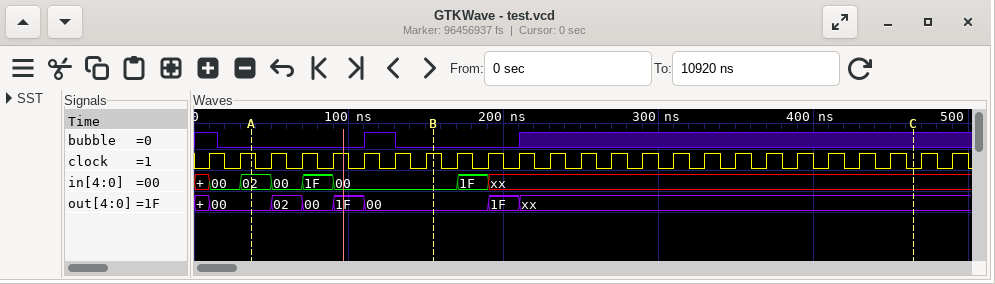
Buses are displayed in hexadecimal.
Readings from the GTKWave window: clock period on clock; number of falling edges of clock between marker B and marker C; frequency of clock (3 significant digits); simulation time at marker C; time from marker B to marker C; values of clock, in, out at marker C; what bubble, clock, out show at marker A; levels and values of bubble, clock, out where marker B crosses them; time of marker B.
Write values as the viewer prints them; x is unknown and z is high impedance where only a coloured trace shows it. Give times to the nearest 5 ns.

20 ns
16
50.0 MHz
465 ns
310 ns
clock=0, in=xx, out=xx
bubble=0, clock=1, out=00
bubble=0, clock=1, out=00
155 ns
